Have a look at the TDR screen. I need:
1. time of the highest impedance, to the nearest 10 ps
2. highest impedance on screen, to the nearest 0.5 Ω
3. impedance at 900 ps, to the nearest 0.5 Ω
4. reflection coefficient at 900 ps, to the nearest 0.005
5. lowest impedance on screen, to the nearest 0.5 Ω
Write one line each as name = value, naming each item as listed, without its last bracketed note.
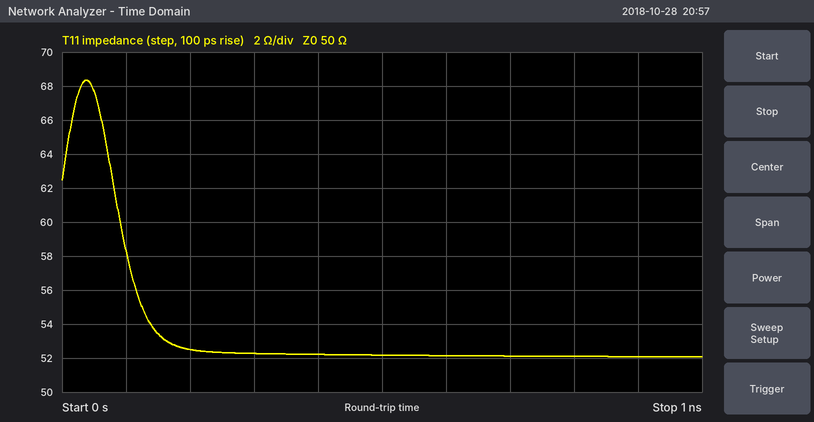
time of the highest impedance, to the nearest 10 ps = 40 ps
highest impedance on screen, to the nearest 0.5 Ω = 68.5 Ω
impedance at 900 ps, to the nearest 0.5 Ω = 52.0 Ω
reflection coefficient at 900 ps, to the nearest 0.005 = +0.020
lowest impedance on screen, to the nearest 0.5 Ω = 52.0 Ω
